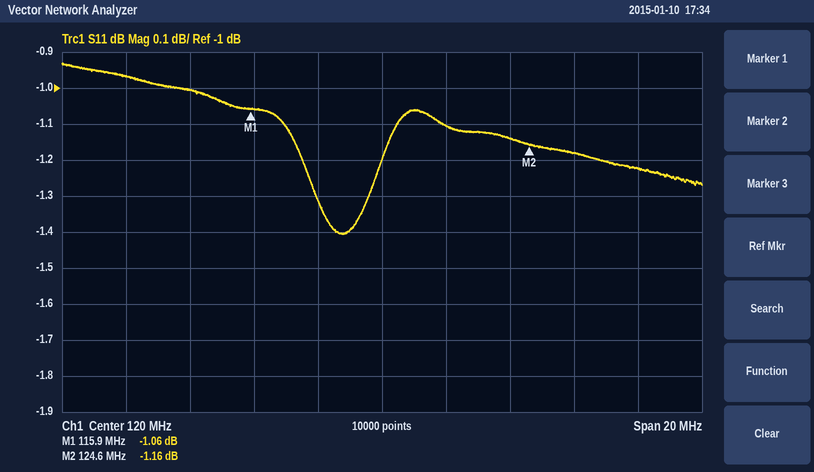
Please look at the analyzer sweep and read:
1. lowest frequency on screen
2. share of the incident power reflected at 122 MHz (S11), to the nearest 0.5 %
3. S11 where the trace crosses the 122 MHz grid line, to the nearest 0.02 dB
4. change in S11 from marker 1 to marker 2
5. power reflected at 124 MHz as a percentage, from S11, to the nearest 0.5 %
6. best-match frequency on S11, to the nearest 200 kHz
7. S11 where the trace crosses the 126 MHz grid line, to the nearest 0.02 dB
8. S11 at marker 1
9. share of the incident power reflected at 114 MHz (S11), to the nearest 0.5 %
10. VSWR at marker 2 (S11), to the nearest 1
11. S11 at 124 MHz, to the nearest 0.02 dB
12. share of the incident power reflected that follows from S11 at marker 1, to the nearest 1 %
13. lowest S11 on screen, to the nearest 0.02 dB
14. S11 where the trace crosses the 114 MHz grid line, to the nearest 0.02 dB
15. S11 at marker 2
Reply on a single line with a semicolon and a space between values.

110 MHz; 77.5 %; -1.10 dB; -0.10 dB; 77.0 %; 118.8 MHz; -1.18 dB; -1.06 dB; 79.5 %; 15; -1.14 dB; 78 %; -1.40 dB; -1.00 dB; -1.16 dB
